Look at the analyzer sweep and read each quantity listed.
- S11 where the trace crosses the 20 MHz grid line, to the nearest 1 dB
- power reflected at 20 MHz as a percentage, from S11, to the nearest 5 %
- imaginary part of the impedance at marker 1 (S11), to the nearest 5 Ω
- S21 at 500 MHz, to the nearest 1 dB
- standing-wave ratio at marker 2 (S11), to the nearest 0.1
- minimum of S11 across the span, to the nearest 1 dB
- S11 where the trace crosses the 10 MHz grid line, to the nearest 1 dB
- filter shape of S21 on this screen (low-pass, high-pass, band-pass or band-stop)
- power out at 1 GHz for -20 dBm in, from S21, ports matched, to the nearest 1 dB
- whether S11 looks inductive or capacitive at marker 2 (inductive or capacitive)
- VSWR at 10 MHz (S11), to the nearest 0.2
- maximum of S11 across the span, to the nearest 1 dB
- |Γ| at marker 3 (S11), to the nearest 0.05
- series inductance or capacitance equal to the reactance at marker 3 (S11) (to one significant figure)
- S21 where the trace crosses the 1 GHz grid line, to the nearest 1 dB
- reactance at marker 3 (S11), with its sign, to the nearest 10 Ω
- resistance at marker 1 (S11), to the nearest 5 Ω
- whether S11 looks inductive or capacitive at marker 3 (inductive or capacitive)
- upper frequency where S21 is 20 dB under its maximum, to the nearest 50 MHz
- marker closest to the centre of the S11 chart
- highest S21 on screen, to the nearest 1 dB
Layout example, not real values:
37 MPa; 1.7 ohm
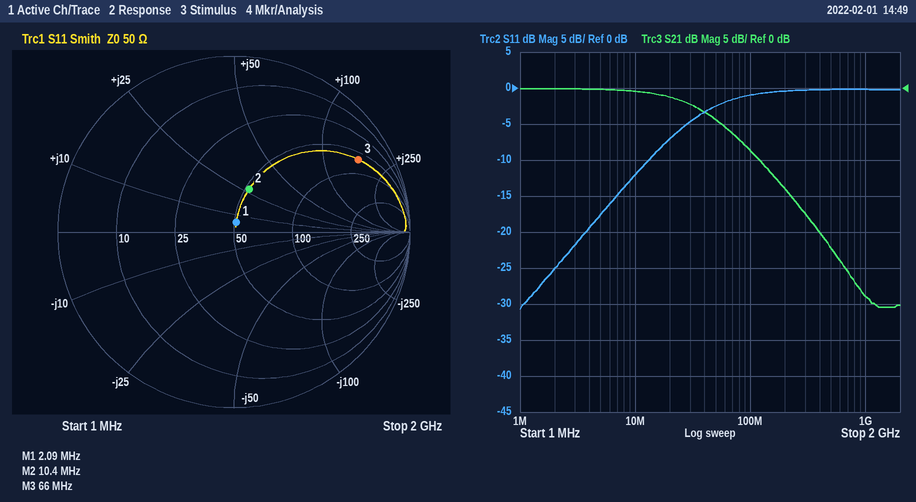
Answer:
-7 dB; 20 %; +5 Ω; -22 dB; 1.7; -31 dB; -12 dB; low-pass; -49 dBm; inductive; 1.6; 0 dB; 0.80; 400 nH; -29 dB; +160 Ω; 50 Ω; inductive; 400 MHz; marker 1; 0 dB
